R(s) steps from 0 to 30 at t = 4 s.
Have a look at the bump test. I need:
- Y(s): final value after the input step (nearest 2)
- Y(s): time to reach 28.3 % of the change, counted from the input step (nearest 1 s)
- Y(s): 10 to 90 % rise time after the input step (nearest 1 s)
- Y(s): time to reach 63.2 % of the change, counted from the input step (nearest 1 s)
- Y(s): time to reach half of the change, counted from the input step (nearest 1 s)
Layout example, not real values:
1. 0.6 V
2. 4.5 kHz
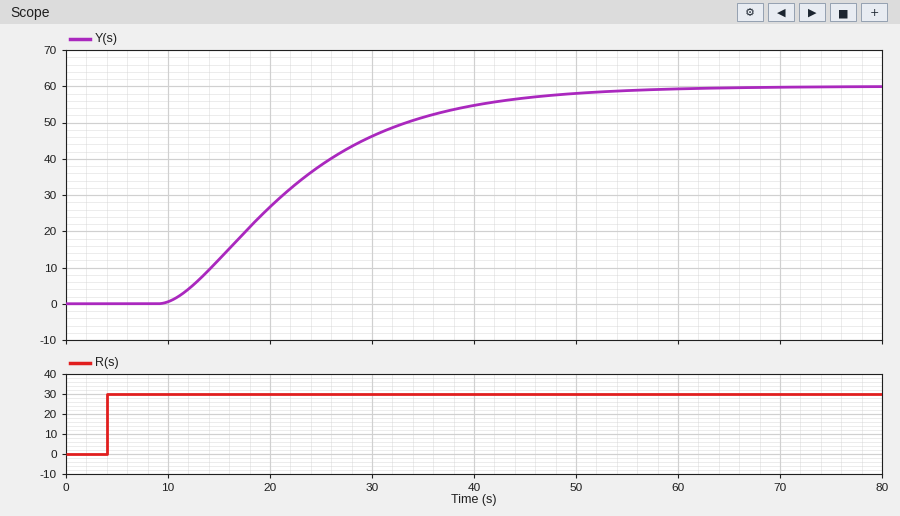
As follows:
1. 60
2. 13 s
3. 26 s
4. 21 s
5. 17 s
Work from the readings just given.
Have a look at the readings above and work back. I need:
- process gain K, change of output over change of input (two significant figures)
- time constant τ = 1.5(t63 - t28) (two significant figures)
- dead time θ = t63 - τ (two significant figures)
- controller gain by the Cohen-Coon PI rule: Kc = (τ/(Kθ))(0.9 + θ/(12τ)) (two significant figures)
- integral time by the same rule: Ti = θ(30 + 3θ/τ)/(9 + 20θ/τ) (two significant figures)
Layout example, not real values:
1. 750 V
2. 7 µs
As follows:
1. 2.0
2. 12 s
3. 9.0 s
4. 0.64
5. 12 s
